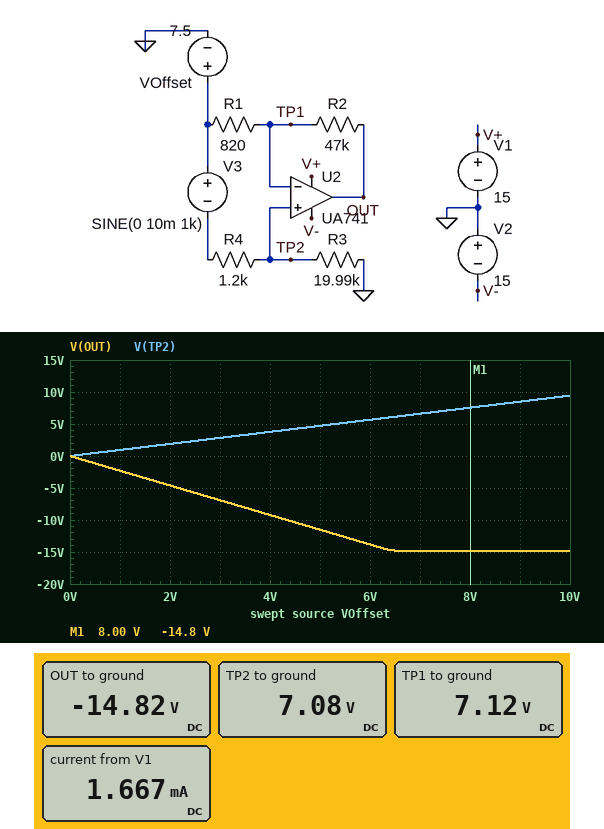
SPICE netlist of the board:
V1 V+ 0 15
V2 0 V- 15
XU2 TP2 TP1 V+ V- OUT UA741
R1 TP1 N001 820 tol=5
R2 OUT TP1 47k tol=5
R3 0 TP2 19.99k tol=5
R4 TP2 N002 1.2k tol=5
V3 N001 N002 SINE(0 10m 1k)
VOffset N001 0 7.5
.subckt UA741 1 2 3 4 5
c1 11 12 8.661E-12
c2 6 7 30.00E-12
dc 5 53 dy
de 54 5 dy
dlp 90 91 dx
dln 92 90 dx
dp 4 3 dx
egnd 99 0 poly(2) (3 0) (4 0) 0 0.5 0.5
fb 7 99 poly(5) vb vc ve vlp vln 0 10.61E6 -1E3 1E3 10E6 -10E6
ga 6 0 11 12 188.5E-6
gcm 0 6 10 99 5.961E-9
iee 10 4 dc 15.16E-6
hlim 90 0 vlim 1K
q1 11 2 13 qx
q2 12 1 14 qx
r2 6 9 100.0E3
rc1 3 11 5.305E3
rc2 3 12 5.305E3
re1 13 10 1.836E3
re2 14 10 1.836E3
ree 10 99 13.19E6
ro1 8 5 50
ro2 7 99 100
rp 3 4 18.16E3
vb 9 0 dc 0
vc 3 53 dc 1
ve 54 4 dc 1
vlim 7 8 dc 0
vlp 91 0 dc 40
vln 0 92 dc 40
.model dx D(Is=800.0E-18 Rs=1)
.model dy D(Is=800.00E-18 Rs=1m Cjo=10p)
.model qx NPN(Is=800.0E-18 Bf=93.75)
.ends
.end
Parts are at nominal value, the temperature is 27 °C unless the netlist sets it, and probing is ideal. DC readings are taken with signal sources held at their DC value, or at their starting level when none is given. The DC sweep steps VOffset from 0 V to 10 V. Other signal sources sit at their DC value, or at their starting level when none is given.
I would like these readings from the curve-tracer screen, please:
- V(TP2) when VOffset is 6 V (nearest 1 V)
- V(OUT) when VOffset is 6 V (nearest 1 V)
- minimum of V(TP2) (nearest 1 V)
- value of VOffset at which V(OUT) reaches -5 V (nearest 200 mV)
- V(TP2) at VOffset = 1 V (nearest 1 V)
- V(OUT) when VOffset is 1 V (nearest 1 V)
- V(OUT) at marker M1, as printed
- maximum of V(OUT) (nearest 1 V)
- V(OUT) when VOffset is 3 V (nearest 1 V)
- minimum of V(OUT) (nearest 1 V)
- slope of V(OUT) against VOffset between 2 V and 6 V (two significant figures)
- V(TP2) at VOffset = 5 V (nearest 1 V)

6 V
-14 V
0 V
2.2 V
1 V
-2 V
-14.8 V
0 V
-7 V
-15 V
-2.3 V/V
5 V
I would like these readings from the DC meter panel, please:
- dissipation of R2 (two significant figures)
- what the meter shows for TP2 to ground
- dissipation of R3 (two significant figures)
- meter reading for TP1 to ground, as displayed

10 mW
7.08 V
2.5 mW
7.12 V
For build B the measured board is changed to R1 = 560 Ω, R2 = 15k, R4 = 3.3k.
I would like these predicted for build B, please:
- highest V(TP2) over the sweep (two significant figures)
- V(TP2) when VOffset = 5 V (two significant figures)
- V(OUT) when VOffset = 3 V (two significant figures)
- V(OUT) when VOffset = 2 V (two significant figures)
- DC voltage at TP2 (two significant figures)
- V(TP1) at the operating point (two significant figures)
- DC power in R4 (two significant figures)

8.6 V
4.3 V
-8.8 V
-5.9 V
6.4 V
6.7 V
340 µW
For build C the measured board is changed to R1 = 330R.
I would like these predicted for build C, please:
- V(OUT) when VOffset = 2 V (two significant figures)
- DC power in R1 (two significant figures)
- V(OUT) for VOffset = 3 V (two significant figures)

-14 V
73 µW
-15 V
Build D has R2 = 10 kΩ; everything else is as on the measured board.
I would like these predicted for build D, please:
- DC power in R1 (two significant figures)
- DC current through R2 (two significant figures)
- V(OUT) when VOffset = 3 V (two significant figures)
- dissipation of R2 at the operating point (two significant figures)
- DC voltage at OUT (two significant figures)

220 µW
520 µA
760 mV
2.7 mW
1.9 V
